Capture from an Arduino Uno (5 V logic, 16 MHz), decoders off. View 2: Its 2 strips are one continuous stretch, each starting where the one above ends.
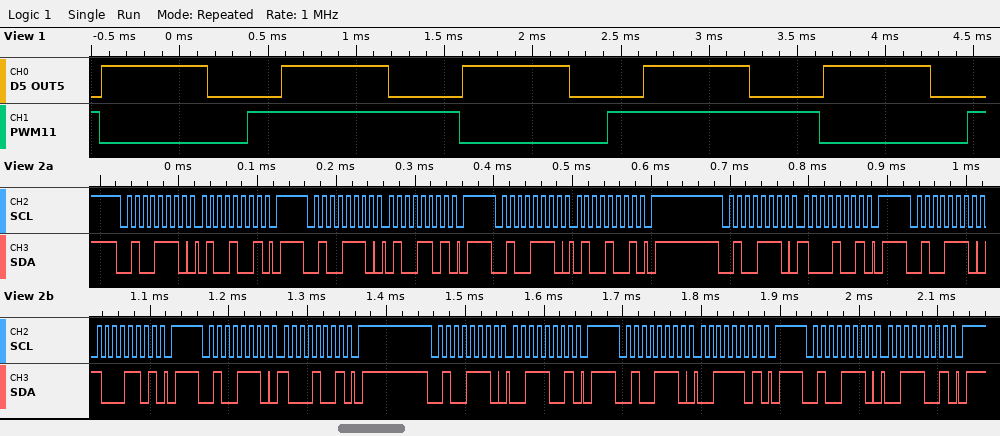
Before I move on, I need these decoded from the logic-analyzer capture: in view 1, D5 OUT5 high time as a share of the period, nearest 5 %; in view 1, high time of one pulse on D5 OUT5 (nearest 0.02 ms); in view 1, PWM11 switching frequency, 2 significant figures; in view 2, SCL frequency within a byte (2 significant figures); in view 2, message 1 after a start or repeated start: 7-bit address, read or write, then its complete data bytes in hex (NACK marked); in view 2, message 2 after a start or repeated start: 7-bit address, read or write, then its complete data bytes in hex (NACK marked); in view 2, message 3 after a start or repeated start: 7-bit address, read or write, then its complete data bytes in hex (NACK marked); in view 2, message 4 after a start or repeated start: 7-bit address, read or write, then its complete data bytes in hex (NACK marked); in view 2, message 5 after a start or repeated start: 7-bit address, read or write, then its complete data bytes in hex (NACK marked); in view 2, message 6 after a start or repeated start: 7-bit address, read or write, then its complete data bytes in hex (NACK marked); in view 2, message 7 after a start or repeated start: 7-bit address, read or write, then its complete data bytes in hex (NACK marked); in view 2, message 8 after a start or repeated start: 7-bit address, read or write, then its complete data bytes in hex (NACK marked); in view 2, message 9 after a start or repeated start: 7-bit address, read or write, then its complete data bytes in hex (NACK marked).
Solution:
60 %
0.60 ms
490 Hz
100 kHz
0x27 write: 49
0x27 write: 4D
0x27 write: 49
0x27 write: 89
0x27 write: 8D
0x27 write: 89
0x27 write: 39
0x27 write: 3D
0x27 write: 39
